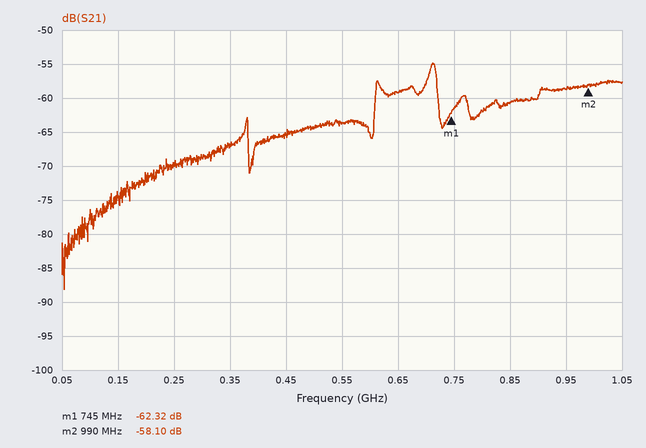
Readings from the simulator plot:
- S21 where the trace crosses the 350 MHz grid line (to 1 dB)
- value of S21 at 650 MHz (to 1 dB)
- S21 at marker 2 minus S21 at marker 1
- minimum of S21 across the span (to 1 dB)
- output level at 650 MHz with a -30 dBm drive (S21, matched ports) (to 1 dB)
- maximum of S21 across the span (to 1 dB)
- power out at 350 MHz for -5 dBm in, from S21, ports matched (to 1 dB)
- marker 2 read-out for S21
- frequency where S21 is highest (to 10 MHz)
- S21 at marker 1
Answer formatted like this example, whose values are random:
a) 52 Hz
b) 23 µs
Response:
a) -67 dB
b) -59 dB
c) 4.22 dB
d) -88 dB
e) -89 dBm
f) -55 dB
g) -72 dBm
h) -58.10 dB
i) 710 MHz
j) -62.32 dB
